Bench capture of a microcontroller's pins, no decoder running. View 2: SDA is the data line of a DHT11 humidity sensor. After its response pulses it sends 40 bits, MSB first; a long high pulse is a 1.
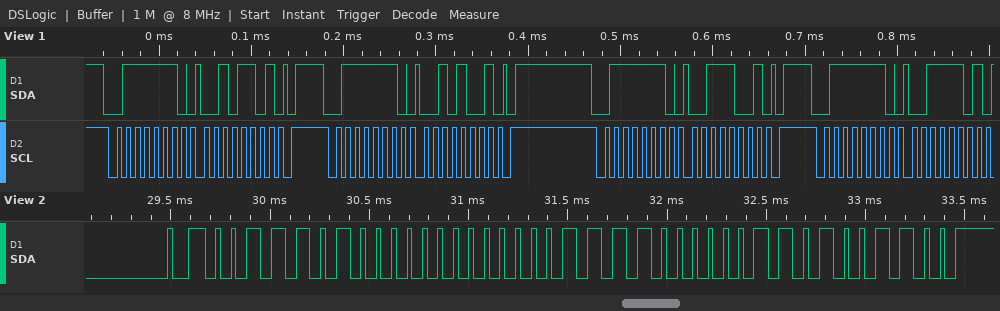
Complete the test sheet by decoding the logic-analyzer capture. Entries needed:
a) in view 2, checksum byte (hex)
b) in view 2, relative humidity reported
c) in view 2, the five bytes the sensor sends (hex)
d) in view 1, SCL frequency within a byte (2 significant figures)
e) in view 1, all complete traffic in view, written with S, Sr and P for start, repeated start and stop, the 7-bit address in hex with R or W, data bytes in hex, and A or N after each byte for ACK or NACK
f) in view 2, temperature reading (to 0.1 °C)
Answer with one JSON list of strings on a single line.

["0x4C", "58 %", "3A 00 0F 03 4C", "100 kHz", "S 3FW A 2D A P S 3FW A 29 A P S 3FW A 39 A P S 3FW A 3D A", "15.3 °C"]
